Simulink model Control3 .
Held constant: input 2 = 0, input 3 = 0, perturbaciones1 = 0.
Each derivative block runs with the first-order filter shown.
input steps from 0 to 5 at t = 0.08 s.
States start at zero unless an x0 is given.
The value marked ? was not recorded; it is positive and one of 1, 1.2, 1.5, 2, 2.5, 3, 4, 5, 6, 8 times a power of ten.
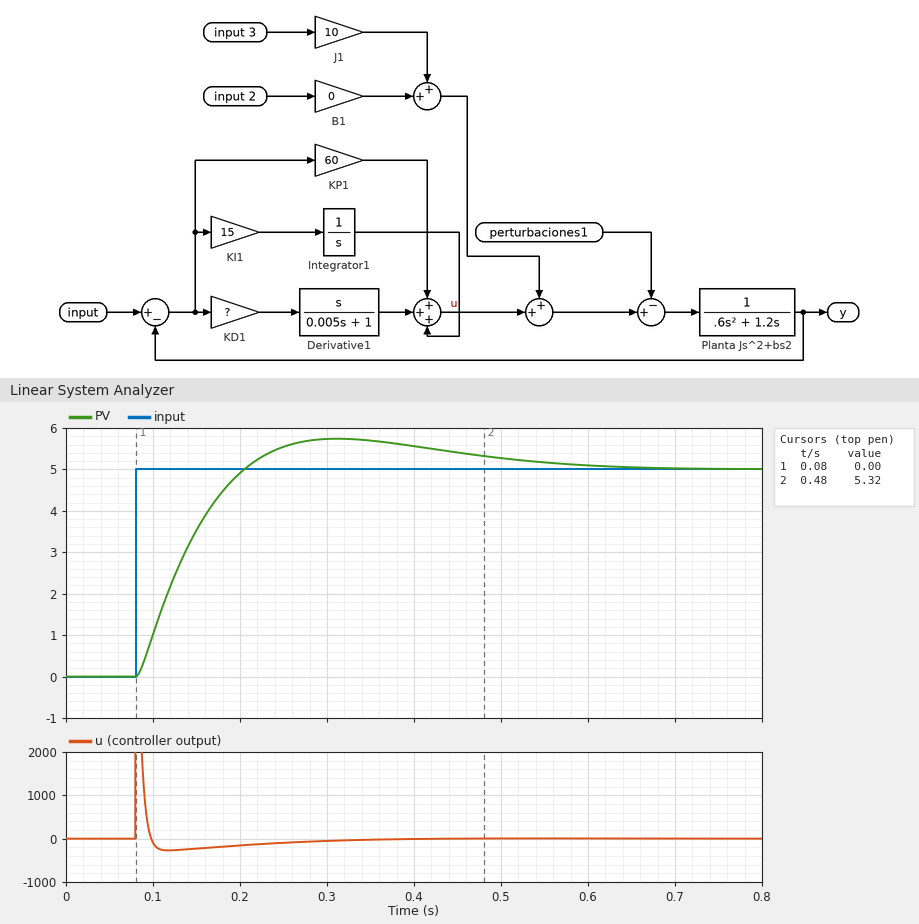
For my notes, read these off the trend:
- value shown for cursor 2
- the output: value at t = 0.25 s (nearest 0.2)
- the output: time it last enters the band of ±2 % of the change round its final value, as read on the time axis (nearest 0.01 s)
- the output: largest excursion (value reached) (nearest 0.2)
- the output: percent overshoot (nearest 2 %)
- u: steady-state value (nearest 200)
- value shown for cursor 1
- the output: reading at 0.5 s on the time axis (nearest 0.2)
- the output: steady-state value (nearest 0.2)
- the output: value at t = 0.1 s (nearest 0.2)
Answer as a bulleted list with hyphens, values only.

- 5.32
- 5.6
- 0.59 s
- 5.8
- 14 %
- 0
- 0.00
- 5.2
- 5.0
- 1.0
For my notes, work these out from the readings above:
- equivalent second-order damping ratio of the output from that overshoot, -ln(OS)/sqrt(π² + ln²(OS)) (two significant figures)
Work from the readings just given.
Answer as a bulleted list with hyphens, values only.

- 0.53
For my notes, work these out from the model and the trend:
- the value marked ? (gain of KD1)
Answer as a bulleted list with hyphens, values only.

- 8
